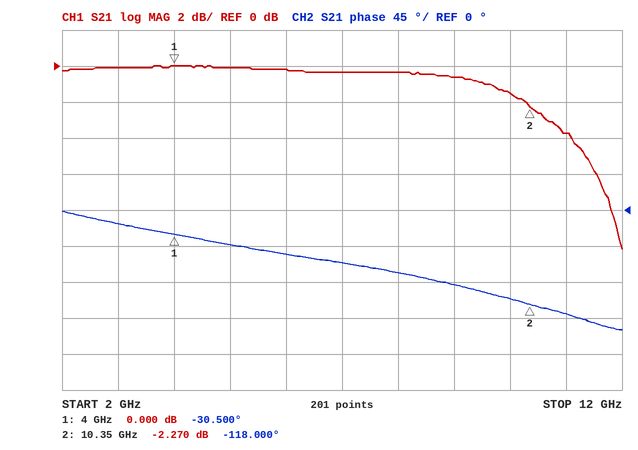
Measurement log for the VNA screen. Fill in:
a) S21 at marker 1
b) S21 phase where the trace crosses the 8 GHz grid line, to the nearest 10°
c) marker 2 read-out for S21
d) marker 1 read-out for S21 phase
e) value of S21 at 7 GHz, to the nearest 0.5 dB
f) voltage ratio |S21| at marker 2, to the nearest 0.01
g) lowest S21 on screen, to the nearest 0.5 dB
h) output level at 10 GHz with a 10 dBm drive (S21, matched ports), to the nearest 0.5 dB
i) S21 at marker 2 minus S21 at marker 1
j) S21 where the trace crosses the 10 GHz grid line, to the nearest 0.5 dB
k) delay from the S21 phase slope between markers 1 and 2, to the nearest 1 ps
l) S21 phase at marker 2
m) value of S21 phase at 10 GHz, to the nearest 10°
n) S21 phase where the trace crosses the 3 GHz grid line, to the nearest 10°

0.000 dB
-80°
-2.270 dB
-30.500°
-0.5 dB
0.77
-10.0 dB
8.5 dBm
-2.270 dB
-1.5 dB
38 ps
-118.000°
-110°
-20°
